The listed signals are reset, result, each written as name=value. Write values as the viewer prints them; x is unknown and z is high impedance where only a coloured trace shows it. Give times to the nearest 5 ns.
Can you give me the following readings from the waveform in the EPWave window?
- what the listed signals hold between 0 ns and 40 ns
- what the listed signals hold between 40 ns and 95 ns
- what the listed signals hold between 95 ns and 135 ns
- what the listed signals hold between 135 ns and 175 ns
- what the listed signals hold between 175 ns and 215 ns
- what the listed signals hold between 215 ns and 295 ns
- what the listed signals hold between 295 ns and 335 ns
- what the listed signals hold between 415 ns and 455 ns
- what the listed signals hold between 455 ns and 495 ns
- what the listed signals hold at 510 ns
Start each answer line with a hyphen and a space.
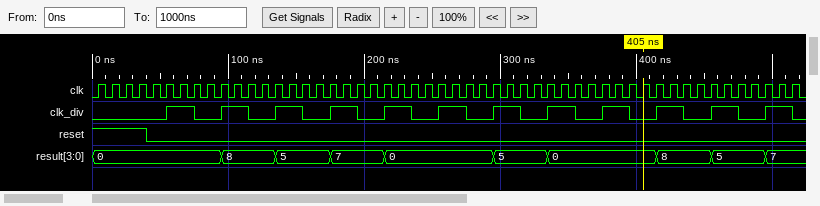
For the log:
- reset=1, result=0
- reset=0, result=0
- reset=0, result=8
- reset=0, result=5
- reset=0, result=7
- reset=0, result=0
- reset=0, result=5
- reset=0, result=8
- reset=0, result=5
- reset=0, result=7
